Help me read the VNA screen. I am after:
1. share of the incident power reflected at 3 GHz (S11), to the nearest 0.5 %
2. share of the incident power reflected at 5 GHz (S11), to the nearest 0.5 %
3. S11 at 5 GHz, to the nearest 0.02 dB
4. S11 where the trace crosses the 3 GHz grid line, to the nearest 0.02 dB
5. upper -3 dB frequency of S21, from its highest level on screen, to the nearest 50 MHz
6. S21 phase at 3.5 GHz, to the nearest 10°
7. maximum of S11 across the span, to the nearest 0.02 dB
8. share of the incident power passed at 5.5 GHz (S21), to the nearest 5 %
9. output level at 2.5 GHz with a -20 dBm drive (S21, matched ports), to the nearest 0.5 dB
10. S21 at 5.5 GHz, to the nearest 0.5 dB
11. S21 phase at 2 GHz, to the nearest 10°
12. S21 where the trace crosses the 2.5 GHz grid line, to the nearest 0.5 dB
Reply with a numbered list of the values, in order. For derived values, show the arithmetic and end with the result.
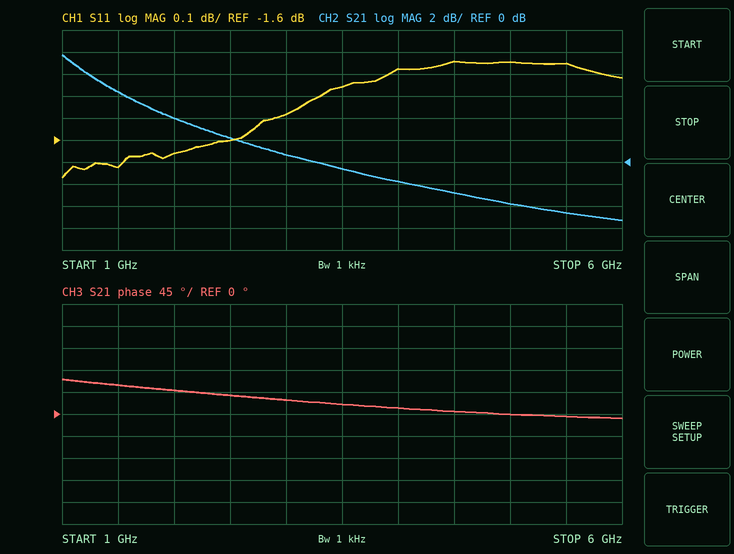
1. 10^(-1.48/10) ≈ 71.1 %, so 71.0 % to the nearest 0.5 %
2. 10^(-1.24/10) ≈ 75.2 %, so 75.0 % to the nearest 0.5 %
3. -1.24 dB
4. -1.48 dB
5. 1.45 GHz
6. 20°
7. -1.24 dB
8. 10^(-4.5/10) ≈ 35 %
9. -20 dBm + (2.0 dB) = -18.0 dBm
10. -4.5 dB
11. 50°
12. 2.0 dB
